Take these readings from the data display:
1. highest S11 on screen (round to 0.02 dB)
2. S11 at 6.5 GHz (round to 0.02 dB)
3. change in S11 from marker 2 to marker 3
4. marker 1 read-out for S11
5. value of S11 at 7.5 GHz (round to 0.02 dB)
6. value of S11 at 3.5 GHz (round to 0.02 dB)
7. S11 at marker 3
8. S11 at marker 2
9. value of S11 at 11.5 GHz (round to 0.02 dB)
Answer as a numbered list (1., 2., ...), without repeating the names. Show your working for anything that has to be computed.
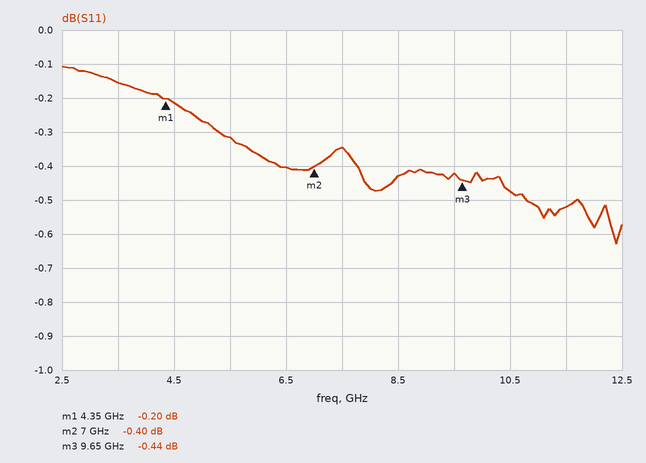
1. -0.10 dB
2. -0.40 dB
3. -0.44 − (-0.4) = -0.04 dB
4. -0.20 dB
5. -0.34 dB
6. -0.16 dB
7. -0.44 dB
8. -0.40 dB
9. -0.52 dB
